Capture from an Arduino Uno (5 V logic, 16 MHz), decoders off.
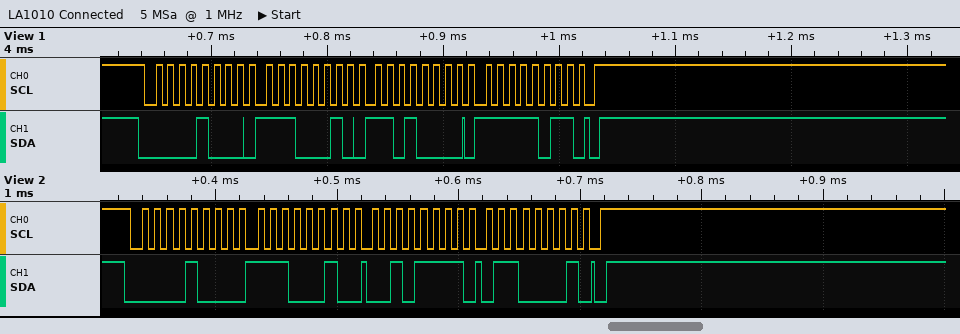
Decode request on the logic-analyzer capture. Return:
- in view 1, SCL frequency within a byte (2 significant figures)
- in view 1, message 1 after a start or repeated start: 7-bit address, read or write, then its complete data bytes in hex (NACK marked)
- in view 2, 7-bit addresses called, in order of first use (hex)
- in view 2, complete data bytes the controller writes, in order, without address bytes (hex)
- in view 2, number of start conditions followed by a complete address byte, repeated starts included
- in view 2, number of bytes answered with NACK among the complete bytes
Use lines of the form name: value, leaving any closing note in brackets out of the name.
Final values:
in view 1, SCL frequency within a byte: 100 kHz
in view 1, message 1 after a start or repeated start: 7-bit address, read or write, then its complete data bytes in hex: 0x04 write: E2 D0 FB
in view 2, 7-bit addresses called, in order of first use: 0x04
in view 2, complete data bytes the controller writes, in order, without address bytes: E2 2F 61
in view 2, number of start conditions followed by a complete address byte, repeated starts included: 1
in view 2, number of bytes answered with NACK among the complete bytes: 0
